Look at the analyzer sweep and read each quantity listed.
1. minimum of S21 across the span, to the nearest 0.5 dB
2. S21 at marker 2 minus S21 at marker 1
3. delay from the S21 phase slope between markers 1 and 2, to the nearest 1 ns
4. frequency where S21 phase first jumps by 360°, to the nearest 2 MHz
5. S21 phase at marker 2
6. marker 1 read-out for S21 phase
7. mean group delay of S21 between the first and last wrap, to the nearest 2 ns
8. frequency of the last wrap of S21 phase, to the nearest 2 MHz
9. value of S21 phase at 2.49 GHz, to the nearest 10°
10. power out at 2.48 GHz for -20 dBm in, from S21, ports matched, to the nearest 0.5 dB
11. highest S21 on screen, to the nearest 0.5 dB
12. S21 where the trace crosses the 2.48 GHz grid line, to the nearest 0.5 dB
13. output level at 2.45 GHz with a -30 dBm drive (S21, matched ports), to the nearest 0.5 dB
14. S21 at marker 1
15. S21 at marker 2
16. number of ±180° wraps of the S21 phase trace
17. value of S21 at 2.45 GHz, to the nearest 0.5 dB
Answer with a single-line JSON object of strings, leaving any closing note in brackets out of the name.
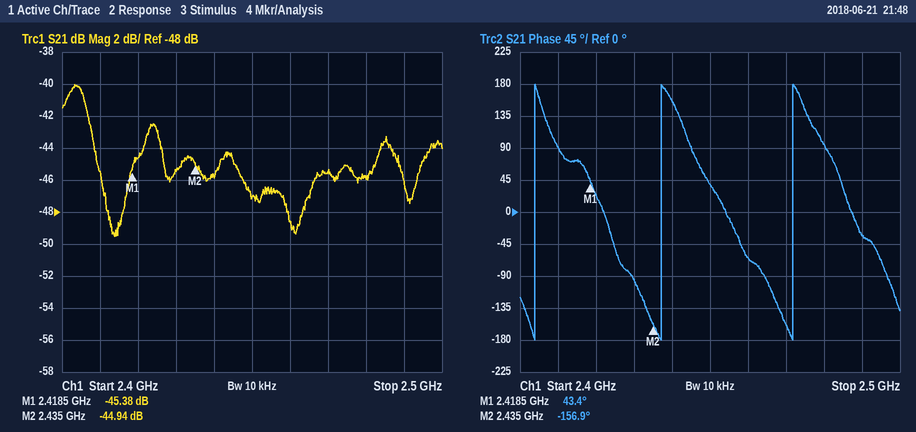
{"minimum of S21 across the span, to the nearest 0.5 dB": "-49.5 dB", "S21 at marker 2 minus S21 at marker 1": "0.44 dB", "delay from the S21 phase slope between markers 1 and 2, to the nearest 1 ns": "34 ns", "frequency where S21 phase first jumps by 360°, to the nearest 2 MHz": "2.404 GHz", "S21 phase at marker 2": "-156.9°", "marker 1 read-out for S21 phase": "43.4°", "mean group delay of S21 between the first and last wrap, to the nearest 2 ns": "30 ns", "frequency of the last wrap of S21 phase, to the nearest 2 MHz": "2.472 GHz", "value of S21 phase at 2.49 GHz, to the nearest 10°": "-30°", "power out at 2.48 GHz for -20 dBm in, from S21, ports matched, to the nearest 0.5 dB": "-66.0 dBm", "highest S21 on screen, to the nearest 0.5 dB": "-40.0 dB", "S21 where the trace crosses the 2.48 GHz grid line, to the nearest 0.5 dB": "-46.0 dB", "output level at 2.45 GHz with a -30 dBm drive (S21, matched ports), to the nearest 0.5 dB": "-77.0 dBm", "S21 at marker 1": "-45.38 dB", "S21 at marker 2": "-44.94 dB", "number of ±180° wraps of the S21 phase trace": "3", "value of S21 at 2.45 GHz, to the nearest 0.5 dB": "-47.0 dB"}
